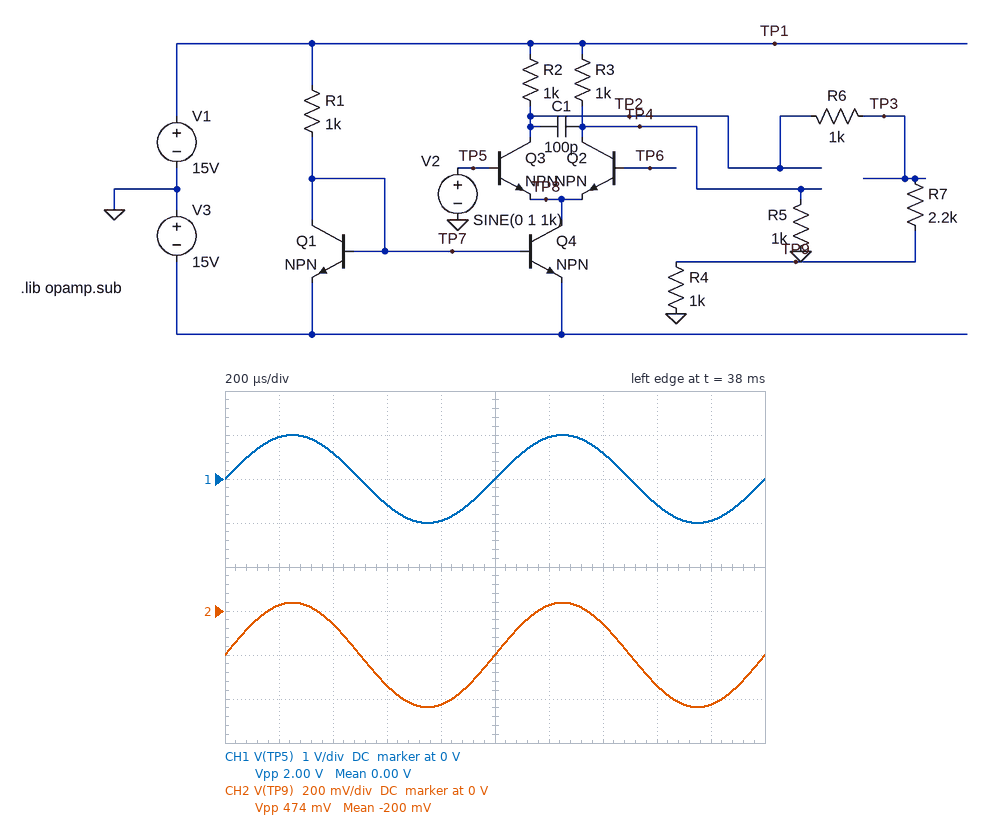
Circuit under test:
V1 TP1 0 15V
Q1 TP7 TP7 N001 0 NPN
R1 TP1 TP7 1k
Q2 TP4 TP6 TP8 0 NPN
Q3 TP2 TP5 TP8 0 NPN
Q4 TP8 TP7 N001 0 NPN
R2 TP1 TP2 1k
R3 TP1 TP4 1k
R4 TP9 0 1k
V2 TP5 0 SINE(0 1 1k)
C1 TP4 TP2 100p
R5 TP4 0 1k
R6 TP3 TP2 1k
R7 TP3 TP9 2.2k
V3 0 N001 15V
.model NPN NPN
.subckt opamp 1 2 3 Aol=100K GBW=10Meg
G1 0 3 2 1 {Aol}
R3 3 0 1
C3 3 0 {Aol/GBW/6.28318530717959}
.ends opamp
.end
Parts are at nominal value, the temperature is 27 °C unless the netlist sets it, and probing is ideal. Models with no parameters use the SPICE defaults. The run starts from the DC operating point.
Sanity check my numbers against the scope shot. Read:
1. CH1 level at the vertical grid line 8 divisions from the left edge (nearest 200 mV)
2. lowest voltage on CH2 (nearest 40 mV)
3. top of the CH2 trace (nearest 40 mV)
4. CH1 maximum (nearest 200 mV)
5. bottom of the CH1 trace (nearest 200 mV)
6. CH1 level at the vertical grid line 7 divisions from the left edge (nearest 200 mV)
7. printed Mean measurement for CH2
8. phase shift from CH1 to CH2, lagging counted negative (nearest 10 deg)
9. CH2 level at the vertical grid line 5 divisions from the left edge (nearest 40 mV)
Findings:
-600 mV
-440 mV
40 mV
1.0 V
-1.0 V
600 mV
-200 mV
0 deg
-200 mV
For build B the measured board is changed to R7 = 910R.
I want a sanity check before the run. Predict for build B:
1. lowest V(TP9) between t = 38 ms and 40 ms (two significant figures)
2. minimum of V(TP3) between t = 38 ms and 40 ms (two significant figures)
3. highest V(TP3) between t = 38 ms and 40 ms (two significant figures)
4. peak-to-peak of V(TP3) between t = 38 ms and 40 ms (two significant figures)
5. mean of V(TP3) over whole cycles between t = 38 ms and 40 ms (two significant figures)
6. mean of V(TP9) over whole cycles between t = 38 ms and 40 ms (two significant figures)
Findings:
-630 mV
-1.2 V
100 mV
1.3 V
-550 mV
-290 mV
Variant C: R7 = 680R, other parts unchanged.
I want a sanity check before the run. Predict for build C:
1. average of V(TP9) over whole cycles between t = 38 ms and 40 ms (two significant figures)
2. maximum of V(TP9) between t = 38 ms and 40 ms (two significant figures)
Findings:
-310 mV
59 mV
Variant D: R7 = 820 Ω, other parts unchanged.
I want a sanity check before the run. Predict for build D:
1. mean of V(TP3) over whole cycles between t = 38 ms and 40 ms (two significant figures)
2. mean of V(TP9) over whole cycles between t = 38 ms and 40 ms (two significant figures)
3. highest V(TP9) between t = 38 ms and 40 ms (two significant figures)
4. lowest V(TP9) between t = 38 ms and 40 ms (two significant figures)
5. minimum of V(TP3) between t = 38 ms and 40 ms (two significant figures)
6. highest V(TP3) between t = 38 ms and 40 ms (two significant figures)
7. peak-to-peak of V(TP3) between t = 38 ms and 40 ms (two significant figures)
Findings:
-540 mV
-300 mV
56 mV
-650 mV
-1.2 V
100 mV
1.3 V
